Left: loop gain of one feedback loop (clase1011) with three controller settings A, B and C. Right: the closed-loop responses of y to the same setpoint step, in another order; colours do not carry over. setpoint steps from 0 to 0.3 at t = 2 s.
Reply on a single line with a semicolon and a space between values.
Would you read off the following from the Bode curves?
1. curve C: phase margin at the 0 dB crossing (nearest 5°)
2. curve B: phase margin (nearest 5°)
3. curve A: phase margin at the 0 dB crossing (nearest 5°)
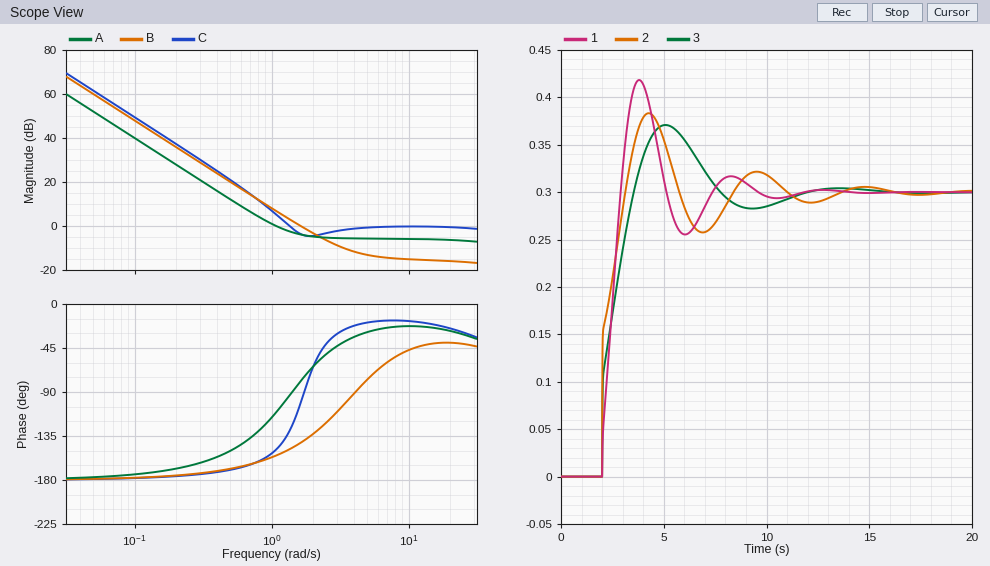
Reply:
50°; 40°; 70°
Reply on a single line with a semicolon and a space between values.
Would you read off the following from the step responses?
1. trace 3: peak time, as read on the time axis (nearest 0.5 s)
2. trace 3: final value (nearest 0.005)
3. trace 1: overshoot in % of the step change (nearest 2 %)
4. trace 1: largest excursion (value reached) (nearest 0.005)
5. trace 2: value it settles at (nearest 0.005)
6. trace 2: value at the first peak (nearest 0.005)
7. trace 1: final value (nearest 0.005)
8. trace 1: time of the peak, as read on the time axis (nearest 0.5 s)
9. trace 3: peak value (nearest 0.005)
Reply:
5.0 s; 0.300; 40 %; 0.420; 0.300; 0.385; 0.300; 4.0 s; 0.370
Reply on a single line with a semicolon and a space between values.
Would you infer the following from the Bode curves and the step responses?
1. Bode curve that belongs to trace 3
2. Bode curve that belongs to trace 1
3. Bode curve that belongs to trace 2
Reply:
A; B; C
